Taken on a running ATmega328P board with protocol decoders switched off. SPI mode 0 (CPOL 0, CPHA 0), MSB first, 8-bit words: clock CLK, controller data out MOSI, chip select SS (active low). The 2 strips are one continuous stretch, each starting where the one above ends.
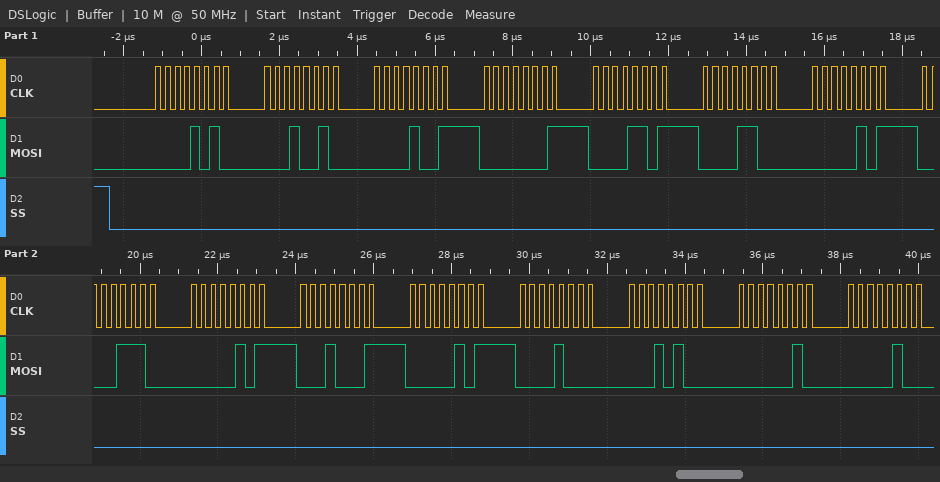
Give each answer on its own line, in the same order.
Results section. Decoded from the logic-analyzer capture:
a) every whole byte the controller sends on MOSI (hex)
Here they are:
0A 12 09 01 0D 0C 05 0E 05 11 05 08 14 02 04
